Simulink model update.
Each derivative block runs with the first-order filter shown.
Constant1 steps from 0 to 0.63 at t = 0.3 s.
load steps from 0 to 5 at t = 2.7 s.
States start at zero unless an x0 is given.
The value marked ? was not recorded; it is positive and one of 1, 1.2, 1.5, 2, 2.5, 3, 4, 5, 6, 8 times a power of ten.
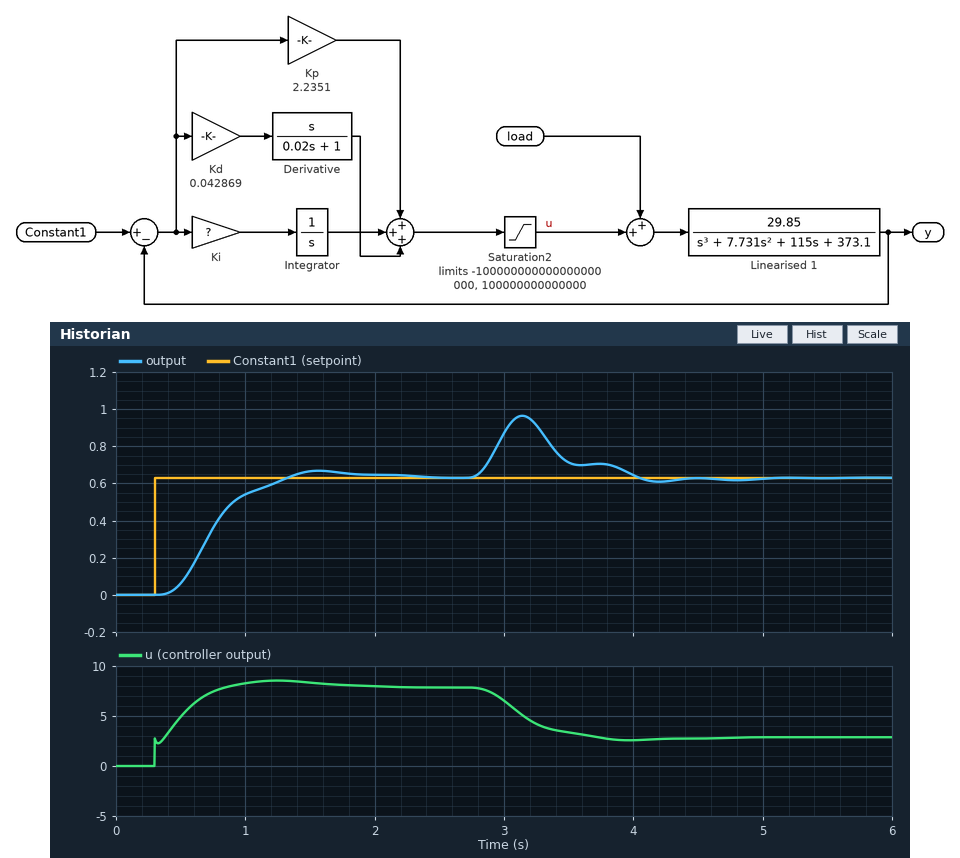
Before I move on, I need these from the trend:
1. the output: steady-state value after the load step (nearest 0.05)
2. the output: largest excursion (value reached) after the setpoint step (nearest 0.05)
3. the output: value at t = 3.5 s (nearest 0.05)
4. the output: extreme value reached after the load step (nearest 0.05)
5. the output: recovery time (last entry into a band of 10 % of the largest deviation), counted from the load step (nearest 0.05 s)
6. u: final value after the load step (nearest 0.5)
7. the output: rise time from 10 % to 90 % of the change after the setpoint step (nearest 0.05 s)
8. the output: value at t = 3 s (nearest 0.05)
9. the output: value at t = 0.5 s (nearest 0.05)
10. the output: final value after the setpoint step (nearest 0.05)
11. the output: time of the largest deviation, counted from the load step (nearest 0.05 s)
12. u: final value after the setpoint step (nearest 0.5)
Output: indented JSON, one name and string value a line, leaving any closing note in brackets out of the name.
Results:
{
  "the output: steady-state value after the load step": "0.65",
  "the output: largest excursion (value reached) after the setpoint step": "0.65",
  "the output: value at t = 3.5 s": "0.70",
  "the output: extreme value reached after the load step": "0.95",
  "the output: recovery time (last entry into a band of 10 % of the largest deviation), counted from the load step": "1.25 s",
  "u: final value after the load step": "3.0",
  "the output: rise time from 10 % to 90 % of the change after the setpoint step": "0.60 s",
  "the output: value at t = 3 s": "0.85",
  "the output: value at t = 0.5 s": "0.05",
  "the output: final value after the setpoint step": "0.65",
  "the output: time of the largest deviation, counted from the load step": "0.45 s",
  "u: final value after the setpoint step": "8.0"
}
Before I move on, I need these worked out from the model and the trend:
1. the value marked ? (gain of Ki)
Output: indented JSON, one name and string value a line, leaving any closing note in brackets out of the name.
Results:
{
  "the value marked ?": "30"
}
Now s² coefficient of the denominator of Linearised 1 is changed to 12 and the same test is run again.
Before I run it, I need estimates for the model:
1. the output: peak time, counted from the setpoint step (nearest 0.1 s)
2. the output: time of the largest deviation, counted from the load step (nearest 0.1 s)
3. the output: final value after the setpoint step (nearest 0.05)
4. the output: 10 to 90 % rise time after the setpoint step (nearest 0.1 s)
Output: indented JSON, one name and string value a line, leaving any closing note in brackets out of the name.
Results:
{
  "the output: peak time, counted from the setpoint step": "1.2 s",
  "the output: time of the largest deviation, counted from the load step": "0.5 s",
  "the output: final value after the setpoint step": "0.65",
  "the output: 10 to 90 % rise time after the setpoint step": "0.5 s"
}
